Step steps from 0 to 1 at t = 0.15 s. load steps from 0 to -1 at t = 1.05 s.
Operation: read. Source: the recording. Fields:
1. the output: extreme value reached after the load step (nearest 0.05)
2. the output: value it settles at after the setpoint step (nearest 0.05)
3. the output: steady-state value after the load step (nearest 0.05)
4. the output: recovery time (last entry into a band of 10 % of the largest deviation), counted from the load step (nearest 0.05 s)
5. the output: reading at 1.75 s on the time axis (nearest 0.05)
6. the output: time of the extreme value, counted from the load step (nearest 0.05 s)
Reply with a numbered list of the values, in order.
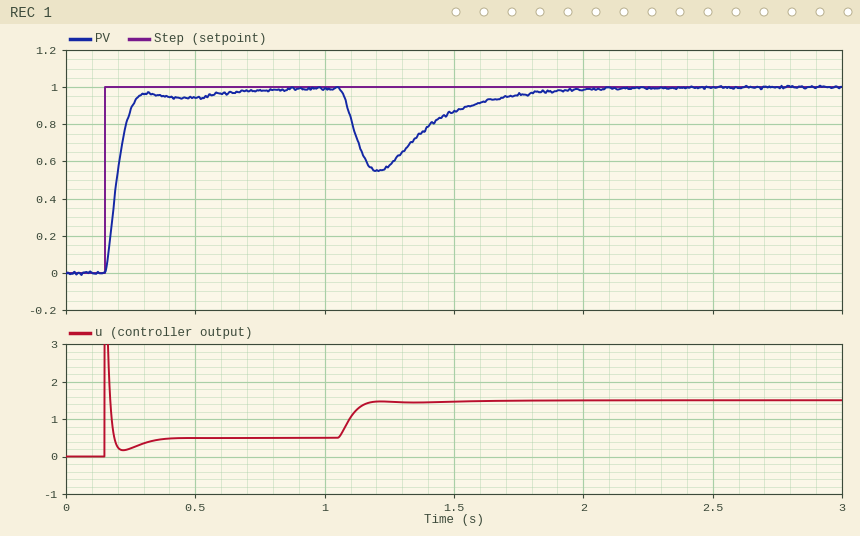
1. 0.55
2. 1.00
3. 1.00
4. 0.70 s
5. 0.95
6. 0.15 s
